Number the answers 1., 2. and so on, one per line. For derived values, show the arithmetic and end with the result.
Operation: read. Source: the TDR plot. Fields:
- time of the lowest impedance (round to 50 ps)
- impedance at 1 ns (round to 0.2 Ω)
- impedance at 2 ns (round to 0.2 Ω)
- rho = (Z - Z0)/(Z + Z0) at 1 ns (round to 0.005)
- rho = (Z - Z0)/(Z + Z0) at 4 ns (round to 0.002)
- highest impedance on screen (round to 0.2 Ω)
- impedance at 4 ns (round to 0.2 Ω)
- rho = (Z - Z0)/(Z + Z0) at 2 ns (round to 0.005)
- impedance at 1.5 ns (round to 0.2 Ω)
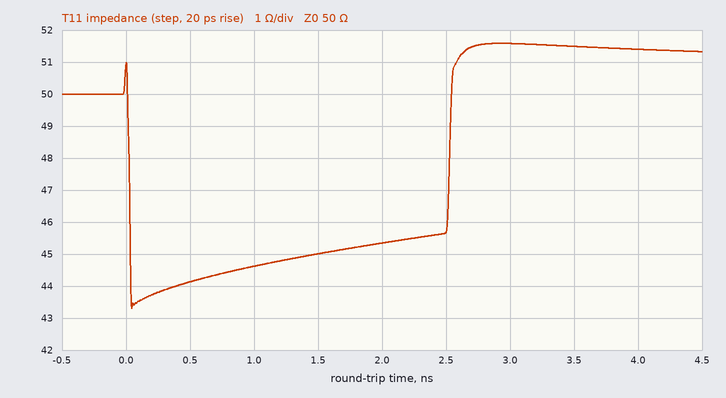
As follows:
1. 50 ps
2. 44.6 Ω
3. 45.4 Ω
4. (44.6 − 50)/(44.6 + 50) ≈ -0.0571, so -0.055 to the nearest 0.005
5. (51.4 − 50)/(51.4 + 50) ≈ +0.014
6. 51.6 Ω
7. 51.4 Ω
8. (45.4 − 50)/(45.4 + 50) ≈ -0.0482, so -0.050 to the nearest 0.005
9. 45.0 Ω
